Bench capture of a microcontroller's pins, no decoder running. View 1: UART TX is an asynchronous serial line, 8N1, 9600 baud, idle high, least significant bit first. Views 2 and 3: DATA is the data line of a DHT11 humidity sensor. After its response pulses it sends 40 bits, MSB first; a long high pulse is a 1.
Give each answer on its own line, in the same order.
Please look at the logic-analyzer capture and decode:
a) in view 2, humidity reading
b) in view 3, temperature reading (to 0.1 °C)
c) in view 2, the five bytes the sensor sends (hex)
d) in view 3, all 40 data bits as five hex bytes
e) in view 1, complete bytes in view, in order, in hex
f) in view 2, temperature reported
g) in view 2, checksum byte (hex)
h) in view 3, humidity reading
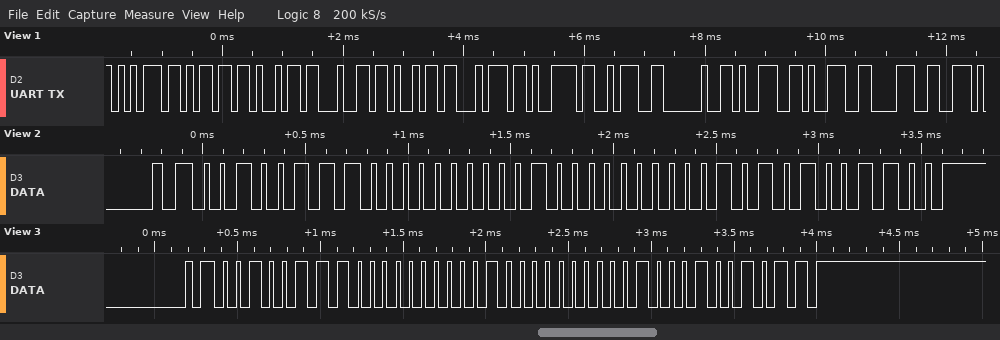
39 %
32.4 °C
27 00 20 05 4C
27 00 20 04 4B
75 6D 69 64 69 74 79 3A 20 39 39 38
32.5 °C
0x4C
39 %
